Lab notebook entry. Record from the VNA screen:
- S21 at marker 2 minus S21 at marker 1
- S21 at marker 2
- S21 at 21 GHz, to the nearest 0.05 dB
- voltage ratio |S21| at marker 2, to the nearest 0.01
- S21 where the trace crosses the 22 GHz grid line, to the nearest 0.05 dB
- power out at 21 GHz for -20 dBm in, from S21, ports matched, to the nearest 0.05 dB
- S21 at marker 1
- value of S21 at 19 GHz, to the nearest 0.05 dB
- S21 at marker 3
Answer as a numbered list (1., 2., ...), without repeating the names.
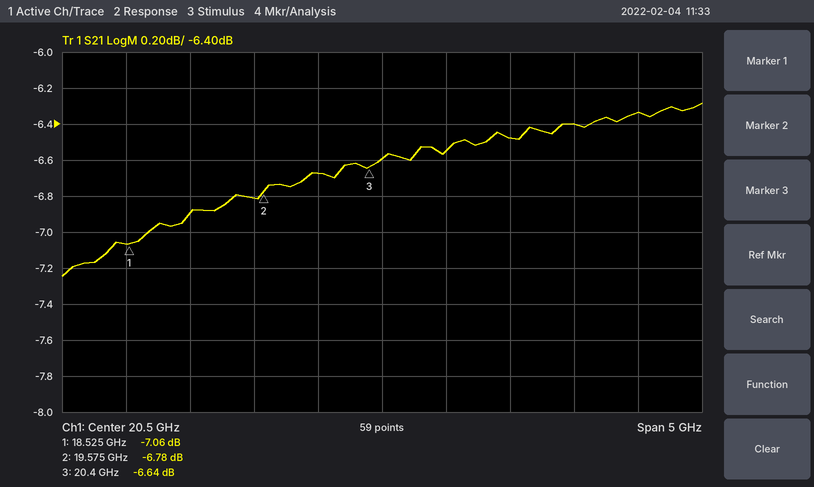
1. 0.28 dB
2. -6.78 dB
3. -6.55 dB
4. 0.46
5. -6.40 dB
6. -26.55 dBm
7. -7.06 dB
8. -6.90 dB
9. -6.64 dB
